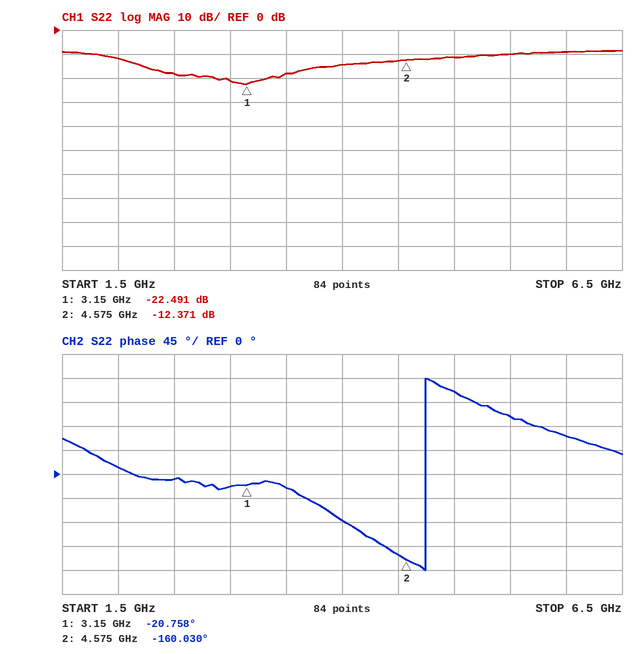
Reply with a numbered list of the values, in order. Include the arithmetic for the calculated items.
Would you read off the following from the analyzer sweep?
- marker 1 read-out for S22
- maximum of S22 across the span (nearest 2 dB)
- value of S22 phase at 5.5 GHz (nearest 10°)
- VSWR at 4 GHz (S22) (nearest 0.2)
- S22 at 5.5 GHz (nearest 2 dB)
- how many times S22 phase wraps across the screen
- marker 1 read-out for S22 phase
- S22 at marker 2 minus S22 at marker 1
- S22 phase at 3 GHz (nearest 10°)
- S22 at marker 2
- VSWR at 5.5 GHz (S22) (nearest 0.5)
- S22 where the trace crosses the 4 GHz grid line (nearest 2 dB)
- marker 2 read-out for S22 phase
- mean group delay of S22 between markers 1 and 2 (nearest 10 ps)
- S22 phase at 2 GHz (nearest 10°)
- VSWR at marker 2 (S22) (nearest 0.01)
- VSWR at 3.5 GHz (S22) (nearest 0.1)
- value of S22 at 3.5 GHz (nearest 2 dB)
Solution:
1. -22.491 dB
2. -8 dB
3. 110°
4. |Γ| = 10^(-14/20) = 0.1995; VSWR = (1 + 0.1995)/(1 − 0.1995) ≈ 1.50, so 1.4 to the nearest 0.2
5. -10 dB
6. 1
7. -20.758°
8. -12.371 − (-22.491) = 10.120 dB
9. -20°
10. -12.371 dB
11. |Γ| = 10^(-10/20) = 0.3162; VSWR = (1 + 0.3162)/(1 − 0.3162) ≈ 1.92, so 2.0 to the nearest 0.5
12. -14 dB
13. -160.030°
14. −(-160.03° − (-20.758°))/(360° × 1.425 GHz) ≈ 271 ps, so 270 ps to the nearest 10 ps
15. 10°
16. (1 + 0.2407)/(1 − 0.2407) ≈ 1.63
17. |Γ| = 10^(-18/20) = 0.1259; VSWR = (1 + 0.1259)/(1 − 0.1259) ≈ 1.3
18. -18 dB
